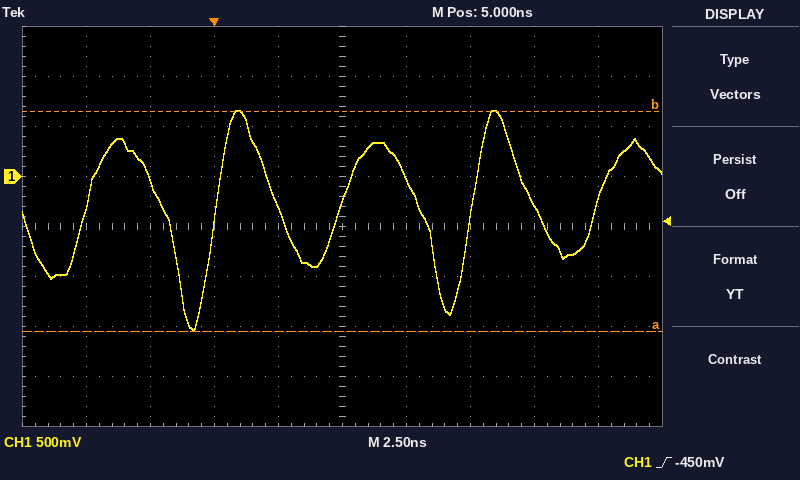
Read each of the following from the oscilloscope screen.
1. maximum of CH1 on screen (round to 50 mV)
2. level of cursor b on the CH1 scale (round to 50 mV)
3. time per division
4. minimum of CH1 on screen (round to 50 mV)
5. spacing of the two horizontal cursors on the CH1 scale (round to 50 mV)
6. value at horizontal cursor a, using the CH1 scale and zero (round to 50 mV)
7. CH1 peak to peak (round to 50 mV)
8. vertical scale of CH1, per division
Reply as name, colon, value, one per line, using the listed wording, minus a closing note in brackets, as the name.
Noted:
maximum of CH1 on screen: 650 mV
level of cursor b on the CH1 scale: 650 mV
time per division: 2.5 ns
minimum of CH1 on screen: -1.55 V
spacing of the two horizontal cursors on the CH1 scale: 2.20 V
value at horizontal cursor a, using the CH1 scale and zero: -1.55 V
CH1 peak to peak: 2.20 V
vertical scale of CH1, per division: 500 mV
